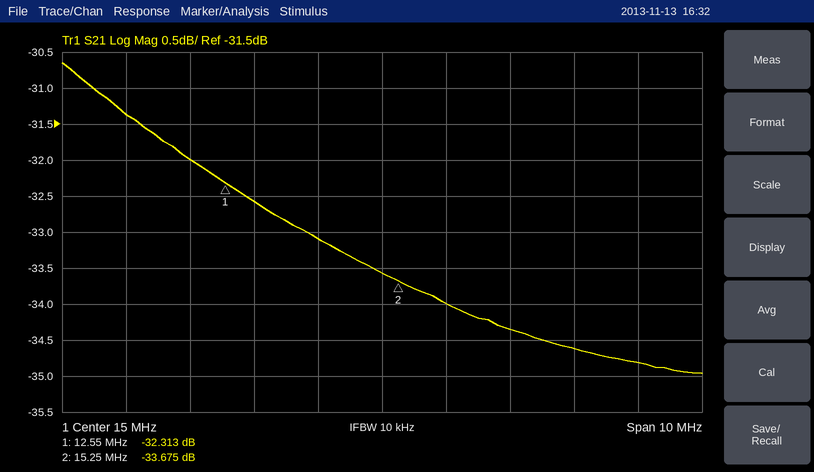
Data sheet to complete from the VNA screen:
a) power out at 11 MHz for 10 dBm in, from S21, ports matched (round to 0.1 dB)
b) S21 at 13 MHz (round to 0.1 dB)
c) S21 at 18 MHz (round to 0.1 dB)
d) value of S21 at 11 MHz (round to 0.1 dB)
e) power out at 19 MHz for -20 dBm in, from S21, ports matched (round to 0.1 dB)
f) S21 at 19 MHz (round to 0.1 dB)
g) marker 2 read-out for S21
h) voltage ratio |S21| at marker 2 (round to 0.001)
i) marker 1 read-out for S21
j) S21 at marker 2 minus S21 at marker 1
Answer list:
-21.4 dBm
-32.6 dB
-34.6 dB
-31.4 dB
-54.8 dBm
-34.8 dB
-33.675 dB
0.021
-32.313 dB
-1.362 dB
